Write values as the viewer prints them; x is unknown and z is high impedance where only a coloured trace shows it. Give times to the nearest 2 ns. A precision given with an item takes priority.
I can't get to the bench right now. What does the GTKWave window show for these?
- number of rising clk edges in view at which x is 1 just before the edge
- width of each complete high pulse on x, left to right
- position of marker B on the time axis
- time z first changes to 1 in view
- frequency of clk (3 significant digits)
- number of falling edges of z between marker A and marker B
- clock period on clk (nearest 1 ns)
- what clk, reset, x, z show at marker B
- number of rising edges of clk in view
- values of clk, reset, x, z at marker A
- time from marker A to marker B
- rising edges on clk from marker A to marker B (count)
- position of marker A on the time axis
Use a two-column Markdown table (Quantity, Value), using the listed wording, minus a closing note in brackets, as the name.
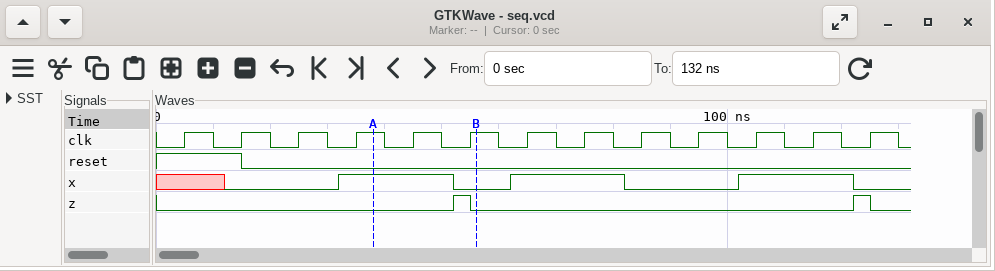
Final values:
| Quantity | Value |
|---|---|
| number of rising clk edges in view at which x is 1 just before the edge | 6 |
| width of each complete high pulse on x, left to right | 20 ns, 20 ns, 20 ns |
| position of marker B on the time axis | 56 ns |
| time z first changes to 1 in view | 52 ns |
| frequency of clk | 100 MHz |
| number of falling edges of z between marker A and marker B | 1 |
| clock period on clk | 10 ns |
| what clk, reset, x, z show at marker B | clk=1, reset=0, x=0, z=0 |
| number of rising edges of clk in view | 13 |
| values of clk, reset, x, z at marker A | clk=1, reset=0, x=1, z=0 |
| time from marker A to marker B | 18 ns |
| rising edges on clk from marker A to marker B | 2 |
| position of marker A on the time axis | 38 ns |
